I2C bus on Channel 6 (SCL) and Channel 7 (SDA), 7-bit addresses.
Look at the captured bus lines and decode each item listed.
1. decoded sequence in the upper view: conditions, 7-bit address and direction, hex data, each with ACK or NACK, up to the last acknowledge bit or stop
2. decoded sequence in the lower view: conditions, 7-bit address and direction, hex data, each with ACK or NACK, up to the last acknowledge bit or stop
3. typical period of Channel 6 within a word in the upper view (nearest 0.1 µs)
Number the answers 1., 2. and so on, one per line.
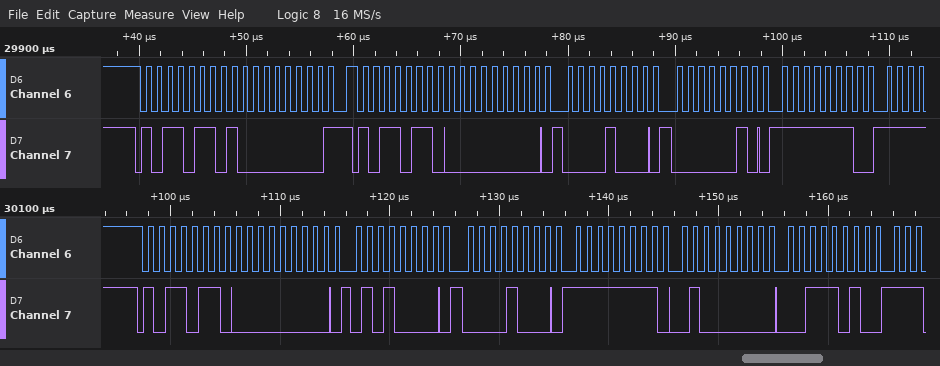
1. start, address 5B write NACK, 00 NACK, repeated start, address 5B write ACK, 00 ACK, 08 ACK, 02 ACK, FE ACK
2. start, address 5B write ACK, 00 ACK, 50 ACK, 08 ACK, FF ACK, 40 ACK, 3A ACK
3. 1 µs
